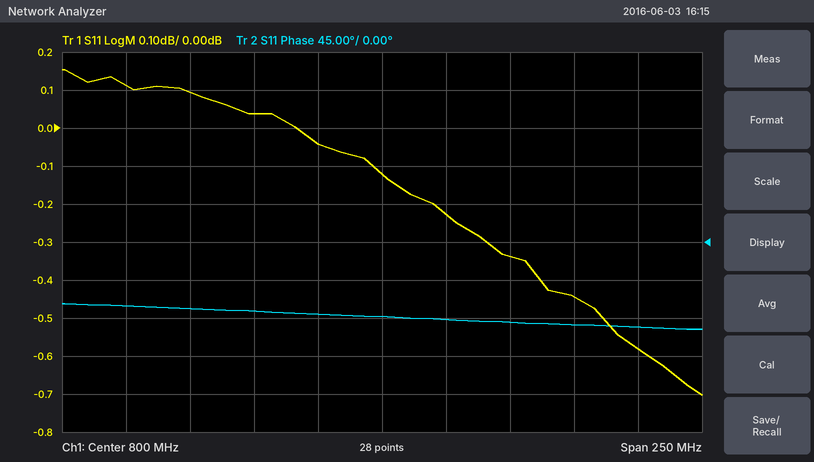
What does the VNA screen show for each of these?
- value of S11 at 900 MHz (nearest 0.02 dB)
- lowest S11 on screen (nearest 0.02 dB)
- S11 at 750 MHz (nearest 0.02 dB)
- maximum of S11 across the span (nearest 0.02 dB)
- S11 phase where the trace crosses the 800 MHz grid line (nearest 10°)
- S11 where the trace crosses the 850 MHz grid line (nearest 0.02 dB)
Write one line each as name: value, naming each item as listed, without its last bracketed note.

value of S11 at 900 MHz: -0.58 dB
lowest S11 on screen: -0.70 dB
S11 at 750 MHz: 0.04 dB
maximum of S11 across the span: 0.16 dB
S11 phase where the trace crosses the 800 MHz grid line: -90°
S11 where the trace crosses the 850 MHz grid line: -0.34 dB
